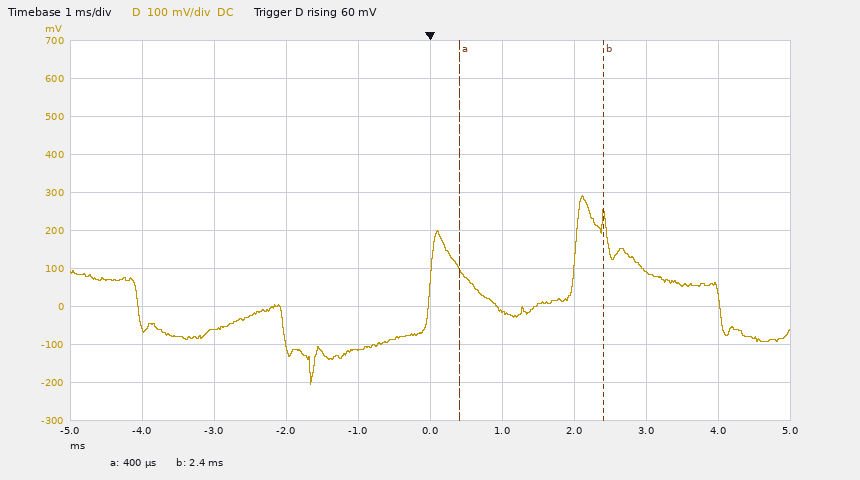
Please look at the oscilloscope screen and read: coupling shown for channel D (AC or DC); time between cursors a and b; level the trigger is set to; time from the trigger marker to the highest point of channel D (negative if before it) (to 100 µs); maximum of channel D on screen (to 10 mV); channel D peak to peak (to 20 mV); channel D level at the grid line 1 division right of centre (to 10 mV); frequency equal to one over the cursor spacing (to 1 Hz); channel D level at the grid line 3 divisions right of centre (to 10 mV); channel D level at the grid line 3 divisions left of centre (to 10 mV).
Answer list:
DC
2.0 ms
60 mV
+2.1 ms
290 mV
500 mV
-10 mV
500 Hz
90 mV
-60 mV
